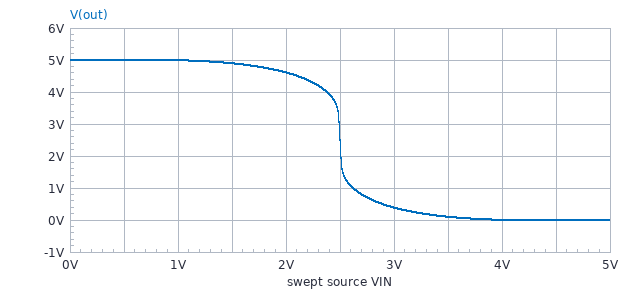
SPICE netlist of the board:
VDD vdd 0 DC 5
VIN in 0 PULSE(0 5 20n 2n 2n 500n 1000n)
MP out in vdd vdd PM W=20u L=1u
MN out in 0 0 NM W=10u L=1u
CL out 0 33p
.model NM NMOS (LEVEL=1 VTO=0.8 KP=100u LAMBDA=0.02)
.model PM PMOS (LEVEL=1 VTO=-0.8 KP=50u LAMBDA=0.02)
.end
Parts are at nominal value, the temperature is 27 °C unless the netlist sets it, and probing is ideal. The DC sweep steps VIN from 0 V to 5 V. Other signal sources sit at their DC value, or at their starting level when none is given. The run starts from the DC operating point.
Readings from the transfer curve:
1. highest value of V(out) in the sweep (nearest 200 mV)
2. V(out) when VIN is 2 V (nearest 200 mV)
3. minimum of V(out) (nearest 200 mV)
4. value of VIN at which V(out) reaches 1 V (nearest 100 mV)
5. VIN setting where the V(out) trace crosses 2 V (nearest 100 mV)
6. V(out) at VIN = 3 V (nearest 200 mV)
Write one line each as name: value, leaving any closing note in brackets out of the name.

highest value of V(out) in the sweep: 5.0 V
V(out) when VIN is 2 V: 4.6 V
minimum of V(out): 0 V
value of VIN at which V(out) reaches 1 V: 2.6 V
VIN setting where the V(out) trace crosses 2 V: 2.5 V
V(out) at VIN = 3 V: 400 mV
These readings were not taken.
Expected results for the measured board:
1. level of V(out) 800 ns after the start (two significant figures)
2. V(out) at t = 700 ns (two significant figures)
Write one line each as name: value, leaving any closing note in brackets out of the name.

level of V(out) 800 ns after the start: 5.0 V
V(out) at t = 700 ns: 5.0 V
